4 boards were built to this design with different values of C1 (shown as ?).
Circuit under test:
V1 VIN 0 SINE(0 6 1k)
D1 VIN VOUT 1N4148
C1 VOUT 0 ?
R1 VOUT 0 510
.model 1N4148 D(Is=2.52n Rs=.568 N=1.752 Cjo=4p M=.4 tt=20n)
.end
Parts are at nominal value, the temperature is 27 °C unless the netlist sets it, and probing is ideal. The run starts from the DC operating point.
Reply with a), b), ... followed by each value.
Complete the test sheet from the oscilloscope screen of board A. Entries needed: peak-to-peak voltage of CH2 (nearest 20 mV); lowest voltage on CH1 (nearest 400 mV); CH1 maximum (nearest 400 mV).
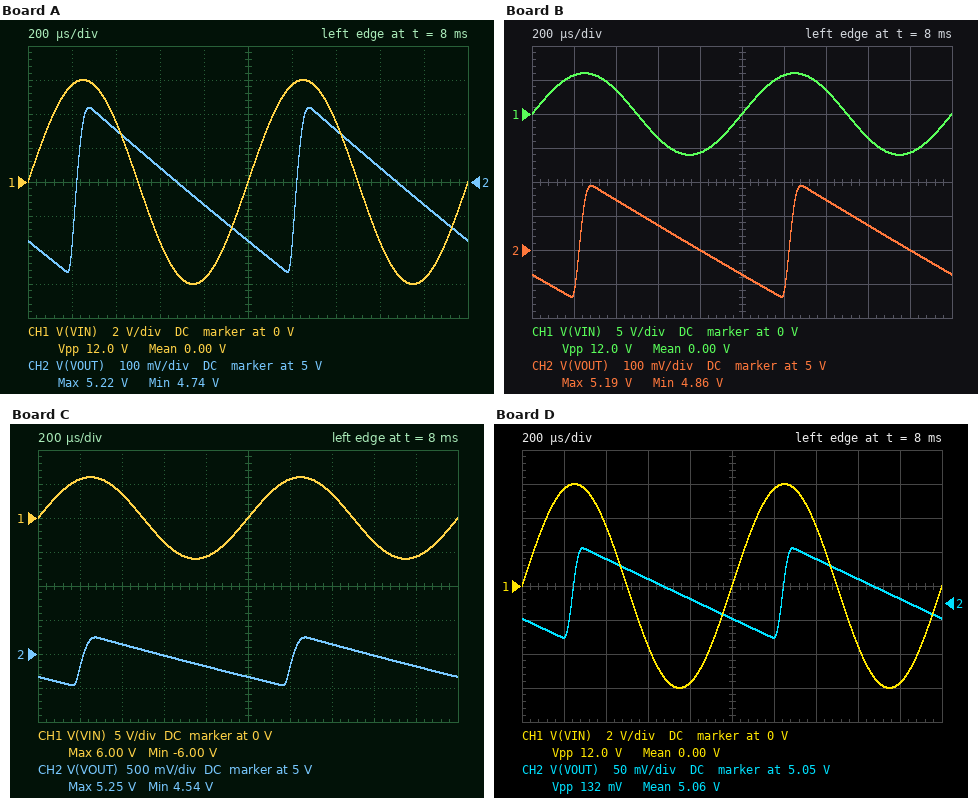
a) 480 mV
b) -6.0 V
c) 6.0 V
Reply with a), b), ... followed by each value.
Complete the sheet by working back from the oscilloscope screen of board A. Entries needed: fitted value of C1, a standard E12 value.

a) 18 µF
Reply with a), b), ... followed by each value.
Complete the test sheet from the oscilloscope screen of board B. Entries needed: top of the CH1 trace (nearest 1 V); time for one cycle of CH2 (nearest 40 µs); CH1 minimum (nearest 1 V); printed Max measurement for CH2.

a) 6 V
b) 1.00 ms
c) -6 V
d) 5.19 V
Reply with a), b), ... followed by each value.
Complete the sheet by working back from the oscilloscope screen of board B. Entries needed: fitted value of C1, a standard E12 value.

a) 27 µF
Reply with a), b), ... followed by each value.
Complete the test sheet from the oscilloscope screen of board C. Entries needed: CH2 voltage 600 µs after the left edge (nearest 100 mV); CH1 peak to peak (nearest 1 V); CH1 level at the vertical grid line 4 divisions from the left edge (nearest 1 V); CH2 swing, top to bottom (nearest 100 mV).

a) 5.0 V
b) 12 V
c) -6 V
d) 700 mV
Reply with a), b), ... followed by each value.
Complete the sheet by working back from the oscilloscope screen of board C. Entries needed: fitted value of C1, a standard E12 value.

a) 12 µF
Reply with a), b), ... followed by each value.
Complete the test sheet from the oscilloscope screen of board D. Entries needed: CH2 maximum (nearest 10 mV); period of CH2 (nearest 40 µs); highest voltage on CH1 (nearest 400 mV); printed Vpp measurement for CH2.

a) 5.13 V
b) 1.00 ms
c) 6.0 V
d) 132 mV
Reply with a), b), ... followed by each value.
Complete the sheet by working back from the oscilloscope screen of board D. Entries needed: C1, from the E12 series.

a) 68 µF
